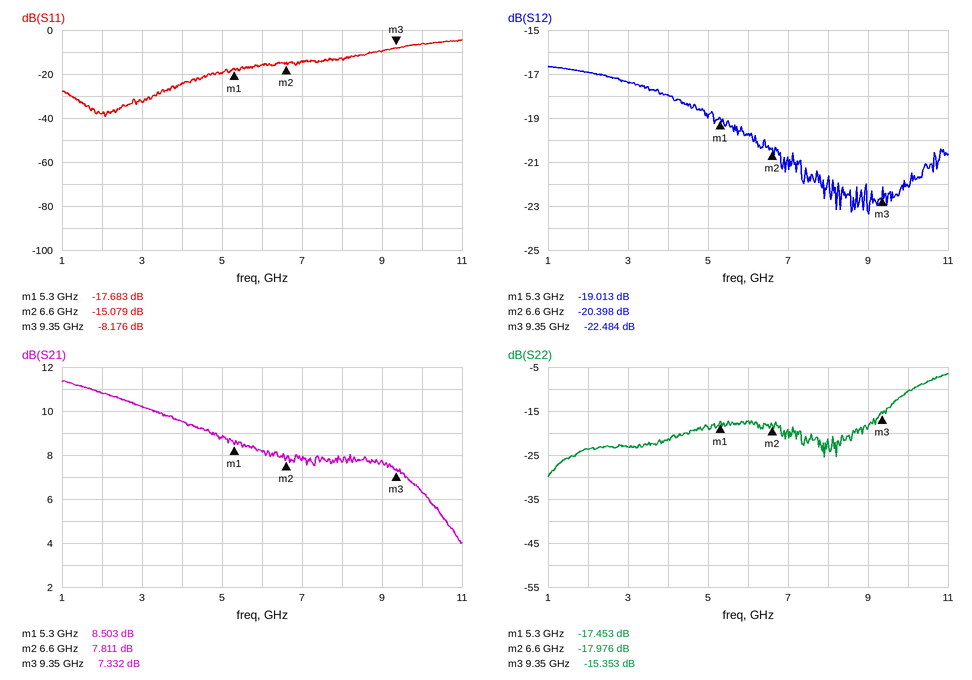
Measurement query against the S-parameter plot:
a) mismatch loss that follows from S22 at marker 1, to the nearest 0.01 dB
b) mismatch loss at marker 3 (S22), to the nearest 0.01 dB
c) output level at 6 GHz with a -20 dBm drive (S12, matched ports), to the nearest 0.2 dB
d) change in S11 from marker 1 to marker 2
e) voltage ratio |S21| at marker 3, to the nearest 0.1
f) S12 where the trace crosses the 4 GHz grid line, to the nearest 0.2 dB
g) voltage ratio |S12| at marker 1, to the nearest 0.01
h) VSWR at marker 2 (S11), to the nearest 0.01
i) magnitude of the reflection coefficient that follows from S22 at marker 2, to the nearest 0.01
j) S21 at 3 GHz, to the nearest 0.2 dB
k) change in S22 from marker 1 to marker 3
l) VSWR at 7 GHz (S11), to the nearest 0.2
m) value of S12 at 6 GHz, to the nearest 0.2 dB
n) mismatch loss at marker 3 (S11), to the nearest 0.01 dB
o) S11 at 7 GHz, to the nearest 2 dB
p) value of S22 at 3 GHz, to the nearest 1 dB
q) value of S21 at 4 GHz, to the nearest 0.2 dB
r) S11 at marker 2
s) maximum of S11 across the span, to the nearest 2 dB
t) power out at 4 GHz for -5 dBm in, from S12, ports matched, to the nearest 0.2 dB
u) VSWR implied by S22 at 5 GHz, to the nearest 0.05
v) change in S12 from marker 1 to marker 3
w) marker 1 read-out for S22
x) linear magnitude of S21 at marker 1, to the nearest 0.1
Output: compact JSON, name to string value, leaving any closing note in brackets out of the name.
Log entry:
{"mismatch loss that follows from S22 at marker 1, to the nearest 0.01 dB": "0.08 dB", "mismatch loss at marker 3 (S22), to the nearest 0.01 dB": "0.13 dB", "output level at 6 GHz with a -20 dBm drive (S12, matched ports), to the nearest 0.2 dB": "-39.8 dBm", "change in S11 from marker 1 to marker 2": "2.604 dB", "voltage ratio |S21| at marker 3, to the nearest 0.1": "2.3", "S12 where the trace crosses the 4 GHz grid line, to the nearest 0.2 dB": "-18.0 dB", "voltage ratio |S12| at marker 1, to the nearest 0.01": "0.11", "VSWR at marker 2 (S11), to the nearest 0.01": "1.43", "magnitude of the reflection coefficient that follows from S22 at marker 2, to the nearest 0.01": "0.13", "S21 at 3 GHz, to the nearest 0.2 dB": "10.2 dB", "change in S22 from marker 1 to marker 3": "2.100 dB", "VSWR at 7 GHz (S11), to the nearest 0.2": "1.4", "value of S12 at 6 GHz, to the nearest 0.2 dB": "-19.8 dB", "mismatch loss at marker 3 (S11), to the nearest 0.01 dB": "0.72 dB", "S11 at 7 GHz, to the nearest 2 dB": "-14 dB", "value of S22 at 3 GHz, to the nearest 1 dB": "-23 dB", "value of S21 at 4 GHz, to the nearest 0.2 dB": "9.6 dB", "S11 at marker 2": "-15.079 dB", "maximum of S11 across the span, to the nearest 2 dB": "-4 dB", "power out at 4 GHz for -5 dBm in, from S12, ports matched, to the nearest 0.2 dB": "-23.0 dBm", "VSWR implied by S22 at 5 GHz, to the nearest 0.05": "1.25", "change in S12 from marker 1 to marker 3": "-3.471 dB", "marker 1 read-out for S22": "-17.453 dB", "linear magnitude of S21 at marker 1, to the nearest 0.1": "2.7"}
